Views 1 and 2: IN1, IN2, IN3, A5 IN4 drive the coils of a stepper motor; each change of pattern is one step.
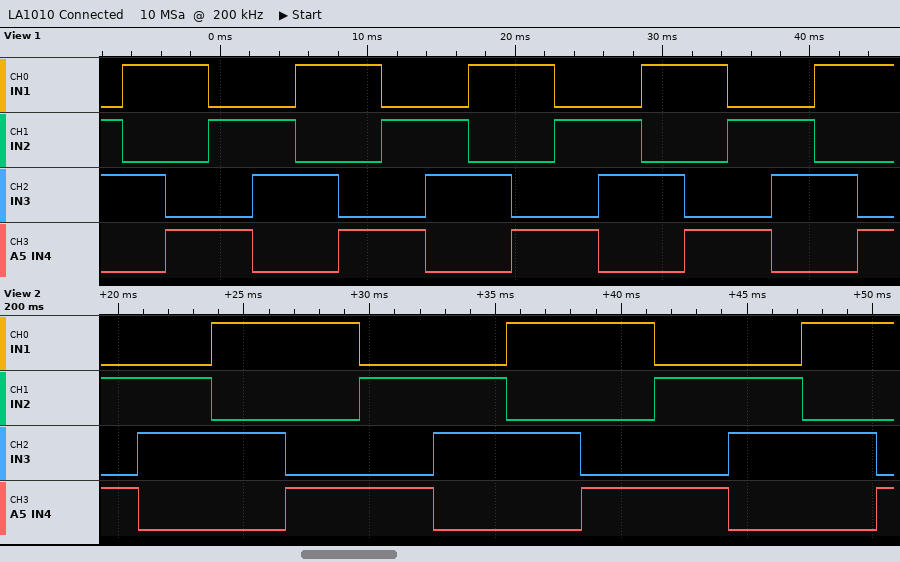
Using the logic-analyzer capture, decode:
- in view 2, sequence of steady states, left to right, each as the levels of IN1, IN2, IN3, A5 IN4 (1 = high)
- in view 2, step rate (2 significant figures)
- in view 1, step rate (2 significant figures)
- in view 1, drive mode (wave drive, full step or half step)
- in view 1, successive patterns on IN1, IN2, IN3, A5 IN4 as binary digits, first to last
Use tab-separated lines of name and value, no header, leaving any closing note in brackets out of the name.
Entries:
in view 2, sequence of steady states, left to right, each as the levels of IN1, IN2, IN3, A5 IN4	0101 0110 1010 1001 0101 0110 1010 1001 0101 0110 1010 1001
in view 2, step rate	340 steps/s
in view 1, step rate	340 steps/s
in view 1, drive mode	full step
in view 1, successive patterns on IN1, IN2, IN3, A5 IN4 as binary digits, first to last	0110 1010 1001 0101 0110 1010 1001 0101 0110 1010 1001 0101 0110 1010 1001 0101 0110 1010 1001
